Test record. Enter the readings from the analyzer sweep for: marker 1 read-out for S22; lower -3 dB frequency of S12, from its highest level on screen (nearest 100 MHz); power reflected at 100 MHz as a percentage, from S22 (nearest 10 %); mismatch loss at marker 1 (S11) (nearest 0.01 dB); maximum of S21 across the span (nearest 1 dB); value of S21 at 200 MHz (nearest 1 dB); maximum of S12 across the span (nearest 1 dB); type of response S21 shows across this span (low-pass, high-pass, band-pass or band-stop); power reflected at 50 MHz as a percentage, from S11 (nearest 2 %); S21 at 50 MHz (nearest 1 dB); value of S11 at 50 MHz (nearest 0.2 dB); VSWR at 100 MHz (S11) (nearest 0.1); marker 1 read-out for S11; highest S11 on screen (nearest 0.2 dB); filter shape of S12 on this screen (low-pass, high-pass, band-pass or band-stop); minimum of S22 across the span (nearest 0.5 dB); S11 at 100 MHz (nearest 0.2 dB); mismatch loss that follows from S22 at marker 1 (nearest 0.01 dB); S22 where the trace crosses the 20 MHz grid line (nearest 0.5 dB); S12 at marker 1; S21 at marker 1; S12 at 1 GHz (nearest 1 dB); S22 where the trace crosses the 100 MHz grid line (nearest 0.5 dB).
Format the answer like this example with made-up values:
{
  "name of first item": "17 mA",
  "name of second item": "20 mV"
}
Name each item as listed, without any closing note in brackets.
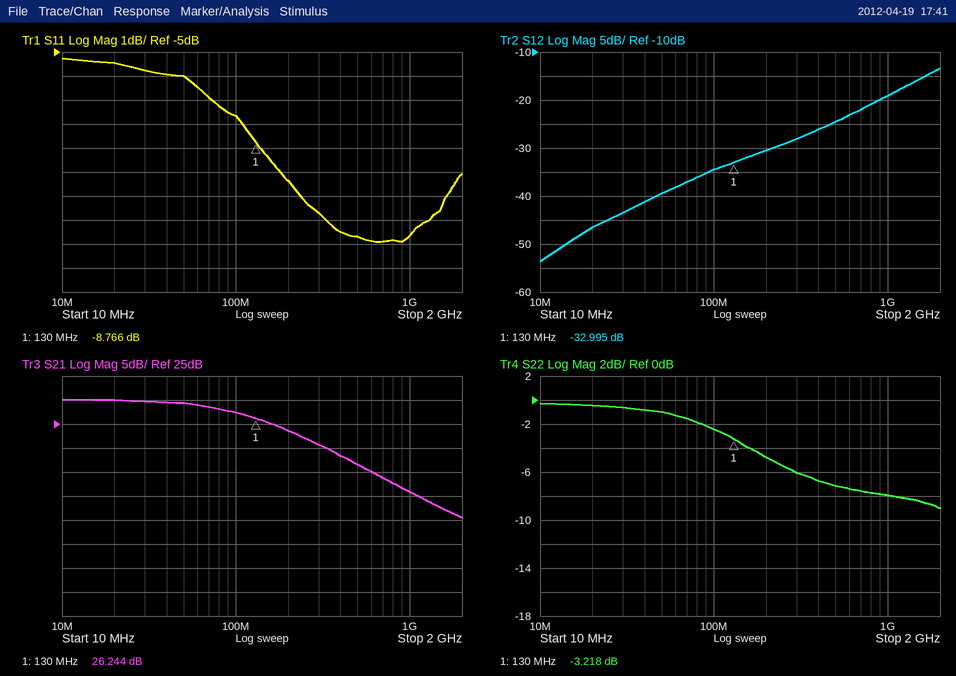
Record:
{
  "marker 1 read-out for S22": "-3.218 dB",
  "lower -3 dB frequency of S12, from its highest level on screen": "1.4 GHz",
  "power reflected at 100 MHz as a percentage, from S22": "60 %",
  "mismatch loss at marker 1 (S11)": "0.62 dB",
  "maximum of S21 across the span": "30 dB",
  "value of S21 at 200 MHz": "24 dB",
  "maximum of S12 across the span": "-13 dB",
  "type of response S21 shows across this span": "low-pass",
  "power reflected at 50 MHz as a percentage, from S11": "26 %",
  "S21 at 50 MHz": "29 dB",
  "value of S11 at 50 MHz": "-6.0 dB",
  "VSWR at 100 MHz (S11)": "2.4",
  "marker 1 read-out for S11": "-8.766 dB",
  "highest S11 on screen": "-5.2 dB",
  "filter shape of S12 on this screen": "high-pass",
  "minimum of S22 across the span": "-9.0 dB",
  "S11 at 100 MHz": "-7.6 dB",
  "mismatch loss that follows from S22 at marker 1": "2.81 dB",
  "S22 where the trace crosses the 20 MHz grid line": "-0.5 dB",
  "S12 at marker 1": "-32.995 dB",
  "S21 at marker 1": "26.244 dB",
  "S12 at 1 GHz": "-19 dB",
  "S22 where the trace crosses the 100 MHz grid line": "-2.5 dB"
}
